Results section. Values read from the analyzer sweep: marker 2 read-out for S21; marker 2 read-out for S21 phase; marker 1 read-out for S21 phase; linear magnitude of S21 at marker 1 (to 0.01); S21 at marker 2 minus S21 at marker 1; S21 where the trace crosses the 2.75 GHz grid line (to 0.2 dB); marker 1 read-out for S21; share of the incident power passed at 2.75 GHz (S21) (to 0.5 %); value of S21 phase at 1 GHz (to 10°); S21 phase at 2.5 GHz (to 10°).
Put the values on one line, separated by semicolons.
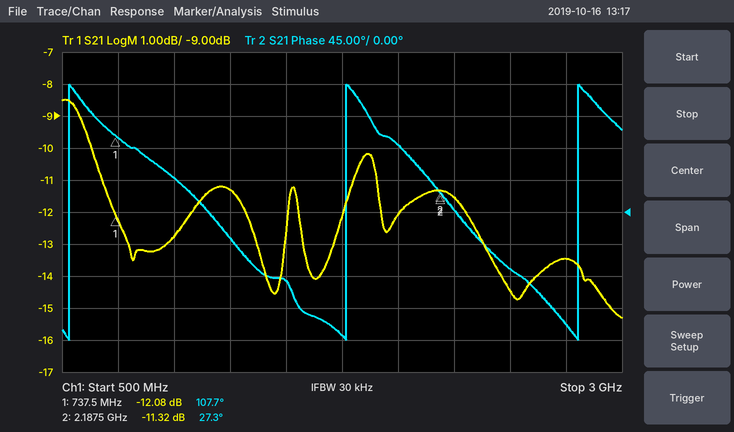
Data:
-11.32 dB; 27.3°; 107.7°; 0.25; 0.76 dB; -13.4 dB; -12.08 dB; 4.5 %; 50°; -80°
